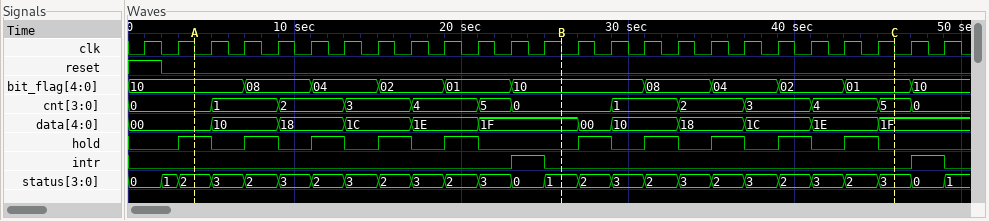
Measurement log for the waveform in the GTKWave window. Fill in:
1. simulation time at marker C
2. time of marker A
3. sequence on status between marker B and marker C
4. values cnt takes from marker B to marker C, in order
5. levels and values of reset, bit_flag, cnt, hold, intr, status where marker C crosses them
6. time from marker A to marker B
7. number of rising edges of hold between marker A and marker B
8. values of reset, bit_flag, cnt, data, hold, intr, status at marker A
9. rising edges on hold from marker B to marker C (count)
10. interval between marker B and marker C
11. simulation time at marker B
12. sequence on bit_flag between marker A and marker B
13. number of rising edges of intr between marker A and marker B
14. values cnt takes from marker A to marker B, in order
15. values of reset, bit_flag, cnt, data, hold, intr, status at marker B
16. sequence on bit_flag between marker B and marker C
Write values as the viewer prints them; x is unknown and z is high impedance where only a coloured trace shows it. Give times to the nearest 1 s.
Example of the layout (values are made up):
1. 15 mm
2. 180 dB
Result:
1. 46 s
2. 4 s
3. 1, 2, 3, 2, 3, 2, 3, 2, 3, 2, 3
4. 0, 1, 2, 3, 4, 5
5. reset=0, bit_flag=01, cnt=5, hold=0, intr=0, status=3
6. 22 s
7. 4
8. reset=0, bit_flag=10, cnt=0, data=00, hold=1, intr=0, status=2
9. 5
10. 20 s
11. 26 s
12. 10, 08, 04, 02, 01, 10
13. 1
14. 0, 1, 2, 3, 4, 5, 0
15. reset=0, bit_flag=10, cnt=0, data=1F, hold=0, intr=0, status=1
16. 10, 08, 04, 02, 01
